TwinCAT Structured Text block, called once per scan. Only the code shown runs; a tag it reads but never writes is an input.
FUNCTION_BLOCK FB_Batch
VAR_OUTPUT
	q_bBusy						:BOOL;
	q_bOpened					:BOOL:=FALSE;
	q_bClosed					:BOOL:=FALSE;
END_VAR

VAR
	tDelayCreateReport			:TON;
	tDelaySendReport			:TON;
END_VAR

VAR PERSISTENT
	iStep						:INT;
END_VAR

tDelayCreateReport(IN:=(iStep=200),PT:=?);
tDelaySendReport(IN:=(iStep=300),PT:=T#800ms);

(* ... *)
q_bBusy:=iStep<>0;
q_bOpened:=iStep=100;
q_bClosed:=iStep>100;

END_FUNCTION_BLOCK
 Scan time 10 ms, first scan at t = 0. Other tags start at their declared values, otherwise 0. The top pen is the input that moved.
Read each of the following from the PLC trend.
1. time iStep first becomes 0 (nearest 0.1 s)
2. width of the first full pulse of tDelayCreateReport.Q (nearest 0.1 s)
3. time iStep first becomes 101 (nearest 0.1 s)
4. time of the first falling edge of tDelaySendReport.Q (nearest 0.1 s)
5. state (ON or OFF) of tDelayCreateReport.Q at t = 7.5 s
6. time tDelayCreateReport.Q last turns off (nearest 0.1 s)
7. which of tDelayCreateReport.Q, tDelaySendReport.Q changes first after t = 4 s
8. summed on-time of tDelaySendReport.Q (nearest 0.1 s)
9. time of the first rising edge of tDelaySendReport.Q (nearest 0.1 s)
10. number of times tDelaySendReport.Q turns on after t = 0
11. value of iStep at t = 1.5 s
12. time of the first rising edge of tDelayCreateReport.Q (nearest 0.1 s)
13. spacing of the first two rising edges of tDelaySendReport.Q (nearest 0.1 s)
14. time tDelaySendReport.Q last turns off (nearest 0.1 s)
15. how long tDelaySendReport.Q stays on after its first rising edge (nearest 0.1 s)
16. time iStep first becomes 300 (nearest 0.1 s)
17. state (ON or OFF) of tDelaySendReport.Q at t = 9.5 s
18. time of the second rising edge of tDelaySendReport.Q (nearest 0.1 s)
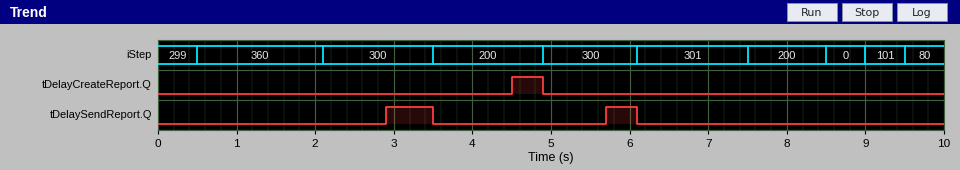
8.5 s
0.4 s
9.0 s
3.5 s
OFF
4.9 s
tDelayCreateReport.Q
1.0 s
2.9 s
2
360
4.5 s
2.8 s
6.1 s
0.6 s
2.1 s
OFF
5.7 s
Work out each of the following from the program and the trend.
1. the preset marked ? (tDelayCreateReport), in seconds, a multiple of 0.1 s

1.0 s
